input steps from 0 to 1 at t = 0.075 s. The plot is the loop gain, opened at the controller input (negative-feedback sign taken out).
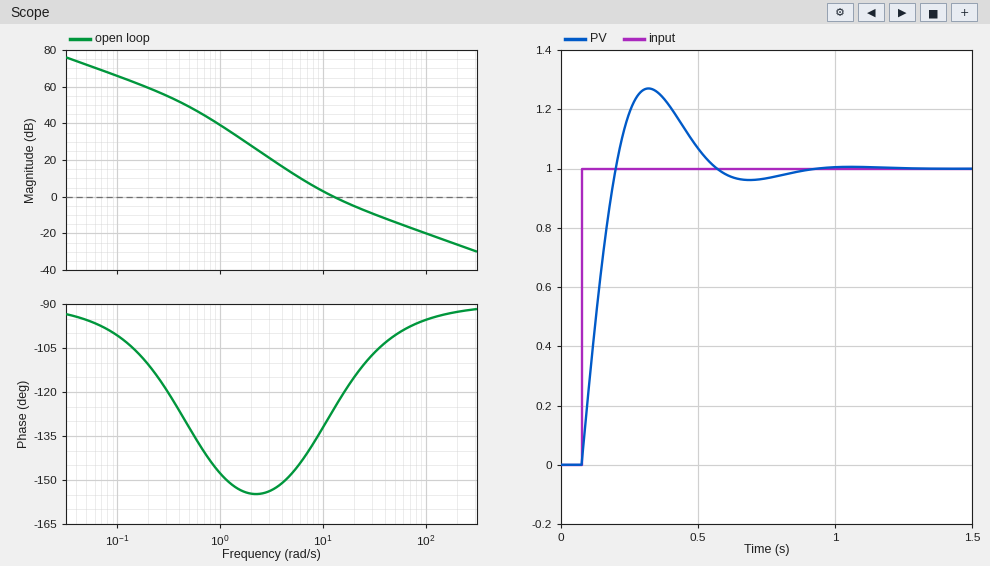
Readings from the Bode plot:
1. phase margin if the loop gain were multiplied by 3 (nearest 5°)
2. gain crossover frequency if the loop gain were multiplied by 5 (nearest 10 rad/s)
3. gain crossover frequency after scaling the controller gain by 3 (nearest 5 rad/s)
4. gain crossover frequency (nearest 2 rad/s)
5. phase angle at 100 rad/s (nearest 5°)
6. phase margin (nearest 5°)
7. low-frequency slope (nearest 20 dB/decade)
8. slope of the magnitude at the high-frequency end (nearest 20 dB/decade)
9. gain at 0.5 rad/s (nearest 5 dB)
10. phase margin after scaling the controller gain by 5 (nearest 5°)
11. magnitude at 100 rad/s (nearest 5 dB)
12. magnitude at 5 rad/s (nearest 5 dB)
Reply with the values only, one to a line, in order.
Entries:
75°
50 rad/s
30 rad/s
12 rad/s
-95°
55°
-20 dB/decade
-20 dB/decade
50 dB
80°
-20 dB
15 dB
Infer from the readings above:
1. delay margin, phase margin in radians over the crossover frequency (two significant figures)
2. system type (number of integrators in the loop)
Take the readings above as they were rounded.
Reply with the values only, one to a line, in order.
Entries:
0.080 s
1
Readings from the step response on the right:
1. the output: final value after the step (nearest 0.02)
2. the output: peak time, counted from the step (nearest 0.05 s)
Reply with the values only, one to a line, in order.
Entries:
1.00
0.25 s
